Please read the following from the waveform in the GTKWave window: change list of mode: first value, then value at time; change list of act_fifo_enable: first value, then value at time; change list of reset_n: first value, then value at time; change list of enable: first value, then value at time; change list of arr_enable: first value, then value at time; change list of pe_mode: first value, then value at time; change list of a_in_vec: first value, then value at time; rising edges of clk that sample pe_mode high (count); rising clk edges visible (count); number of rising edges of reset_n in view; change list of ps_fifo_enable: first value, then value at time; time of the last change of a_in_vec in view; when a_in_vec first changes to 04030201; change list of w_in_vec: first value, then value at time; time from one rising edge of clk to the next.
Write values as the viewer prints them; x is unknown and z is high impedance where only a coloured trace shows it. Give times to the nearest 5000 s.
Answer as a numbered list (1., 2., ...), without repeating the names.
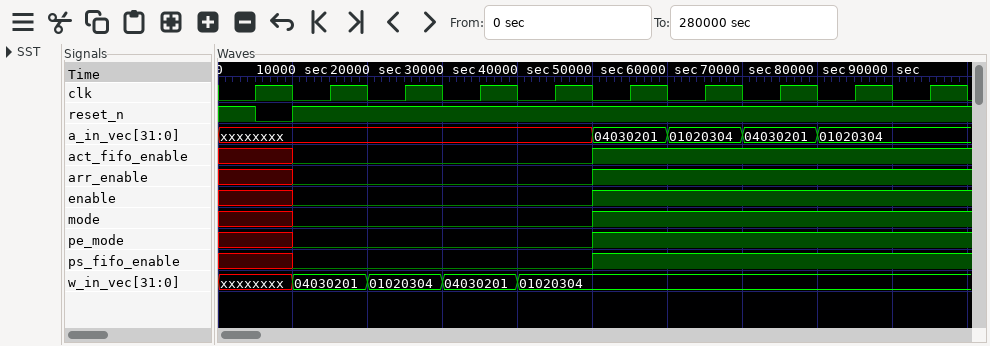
1. x, 0 at 10000 s, 1 at 50000 s
2. x, 0 at 10000 s, 1 at 50000 s
3. 1, 0 at 5000 s, 1 at 10000 s
4. x, 0 at 10000 s, 1 at 50000 s
5. x, 0 at 10000 s, 1 at 50000 s
6. x, 0 at 10000 s, 1 at 50000 s
7. xxxxxxxx, 04030201 at 50000 s, 01020304 at 60000 s, 04030201 at 70000 s, 01020304 at 80000 s
8. 5
9. 10
10. 1
11. x, 0 at 10000 s, 1 at 50000 s
12. 80000 s
13. 50000 s
14. xxxxxxxx, 04030201 at 10000 s, 01020304 at 20000 s, 04030201 at 30000 s, 01020304 at 40000 s
15. 10000 s
